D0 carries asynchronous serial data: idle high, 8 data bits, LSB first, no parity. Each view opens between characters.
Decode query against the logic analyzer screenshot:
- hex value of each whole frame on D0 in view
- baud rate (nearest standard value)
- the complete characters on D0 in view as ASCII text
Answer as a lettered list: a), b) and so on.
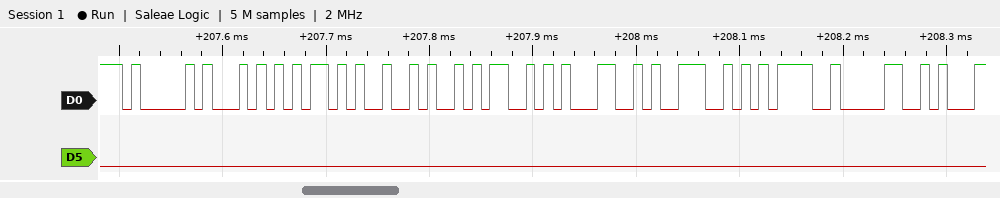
a) 41, 54, 2B, 4A, 53, 4C, 4E, 3D, 30
b) 115200 baud
c) "AT+JSLN=0"
